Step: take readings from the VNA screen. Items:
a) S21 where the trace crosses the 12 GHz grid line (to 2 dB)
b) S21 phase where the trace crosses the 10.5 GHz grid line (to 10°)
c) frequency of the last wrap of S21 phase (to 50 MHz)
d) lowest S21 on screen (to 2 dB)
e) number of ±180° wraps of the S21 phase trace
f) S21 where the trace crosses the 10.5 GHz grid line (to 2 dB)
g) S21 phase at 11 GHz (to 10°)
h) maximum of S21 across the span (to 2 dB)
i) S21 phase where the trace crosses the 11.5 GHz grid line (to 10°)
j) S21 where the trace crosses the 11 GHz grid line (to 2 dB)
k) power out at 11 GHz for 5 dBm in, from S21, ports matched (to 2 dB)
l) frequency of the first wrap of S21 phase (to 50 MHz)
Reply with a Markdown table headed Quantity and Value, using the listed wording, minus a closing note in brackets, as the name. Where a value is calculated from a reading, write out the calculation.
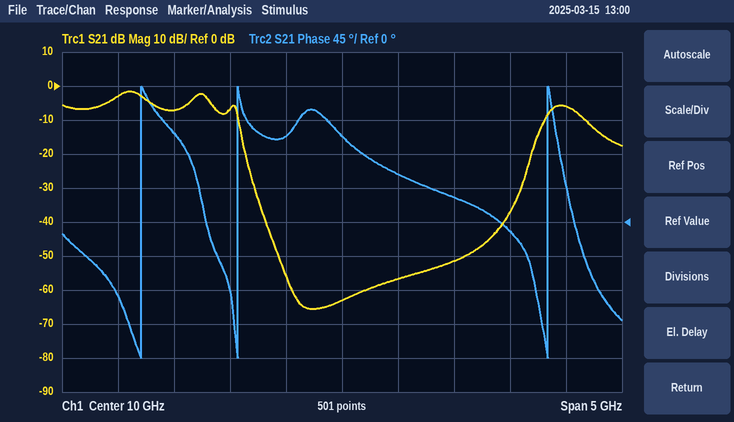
| Quantity | Value |
|---|---|
| S21 where the trace crosses the 12 GHz grid line | -6 dB |
| S21 phase where the trace crosses the 10.5 GHz grid line | 60° |
| frequency of the last wrap of S21 phase | 11.85 GHz |
| lowest S21 on screen | -66 dB |
| number of ±180° wraps of the S21 phase trace | 3 |
| S21 where the trace crosses the 10.5 GHz grid line | -56 dB |
| S21 phase at 11 GHz | 30° |
| maximum of S21 across the span | -2 dB |
| S21 phase where the trace crosses the 11.5 GHz grid line | -10° |
| S21 where the trace crosses the 11 GHz grid line | -52 dB |
| power out at 11 GHz for 5 dBm in, from S21, ports matched | 5 dBm + (-52 dB) = -46 dBm |
| frequency of the first wrap of S21 phase | 8.20 GHz |
